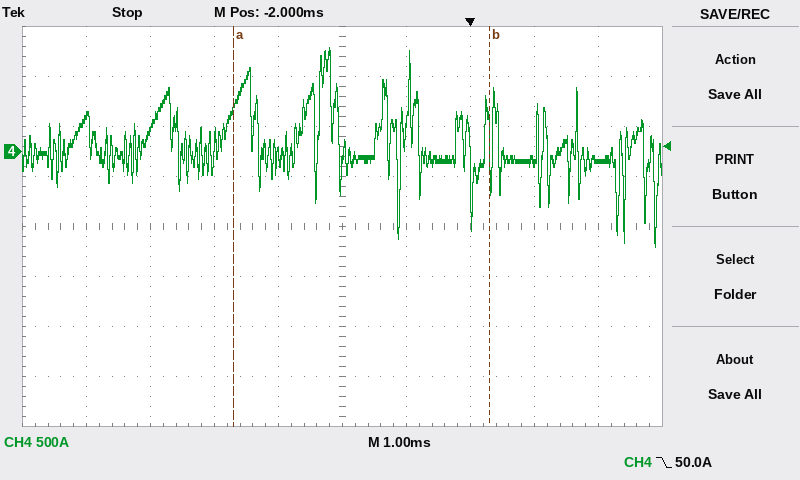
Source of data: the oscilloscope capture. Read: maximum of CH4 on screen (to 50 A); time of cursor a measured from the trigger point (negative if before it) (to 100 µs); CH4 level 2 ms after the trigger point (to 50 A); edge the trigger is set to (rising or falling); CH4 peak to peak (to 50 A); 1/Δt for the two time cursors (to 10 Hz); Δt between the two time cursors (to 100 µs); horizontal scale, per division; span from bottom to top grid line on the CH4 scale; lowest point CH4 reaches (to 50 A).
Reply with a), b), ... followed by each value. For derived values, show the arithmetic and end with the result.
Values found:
a) 1.05 kA
b) -3.7 ms
c) -100 A
d) falling
e) 1.05 kA − (-950 A) = 2.00 kA
f) 1 / 4.0 ms ≈ 250 Hz
g) 4.0 ms
h) 1 ms
i) 4 kA
j) -950 A
